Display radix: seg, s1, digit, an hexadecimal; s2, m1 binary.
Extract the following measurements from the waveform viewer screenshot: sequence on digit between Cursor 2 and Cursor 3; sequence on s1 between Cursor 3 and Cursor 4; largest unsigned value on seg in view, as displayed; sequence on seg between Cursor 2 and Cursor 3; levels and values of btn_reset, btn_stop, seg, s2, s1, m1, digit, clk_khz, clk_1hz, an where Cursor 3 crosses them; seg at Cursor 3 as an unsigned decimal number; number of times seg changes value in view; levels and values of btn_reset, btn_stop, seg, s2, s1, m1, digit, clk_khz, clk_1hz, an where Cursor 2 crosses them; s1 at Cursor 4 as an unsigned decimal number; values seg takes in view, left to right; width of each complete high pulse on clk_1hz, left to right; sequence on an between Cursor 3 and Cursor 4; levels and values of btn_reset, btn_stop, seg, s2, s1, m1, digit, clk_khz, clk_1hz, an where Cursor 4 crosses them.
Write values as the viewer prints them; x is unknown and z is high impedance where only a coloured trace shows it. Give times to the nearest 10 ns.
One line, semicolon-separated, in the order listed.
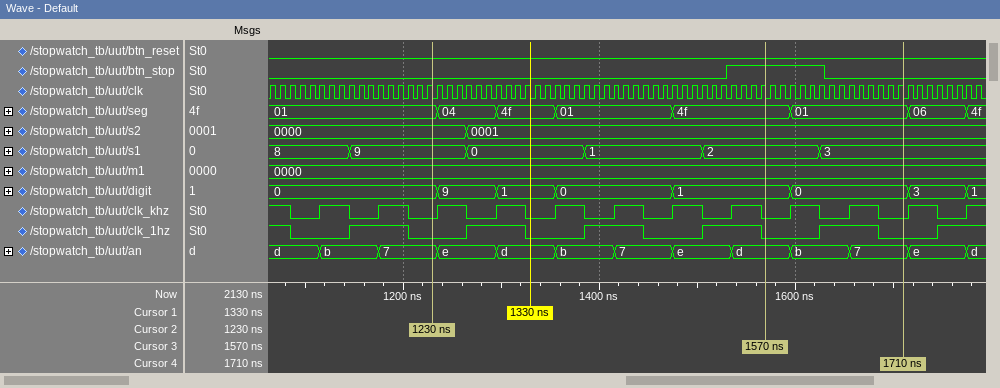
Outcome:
0, 9, 1, 0, 1; 2, 3; 4f; 01, 04, 4f, 01, 4f; btn_reset=0, btn_stop=1, seg=4f, s2=0001, s1=2, m1=0000, digit=1, clk_khz=0, clk_1hz=0, an=d; 79; 7; btn_reset=0, btn_stop=0, seg=01, s2=0000, s1=9, m1=0000, digit=0, clk_khz=0, clk_1hz=0, an=7; 3; 01, 04, 4f, 01, 4f, 01, 06, 4f; 60 ns, 60 ns, 60 ns, 60 ns, 60 ns; d, b, 7; btn_reset=0, btn_stop=0, seg=01, s2=0001, s1=3, m1=0000, digit=0, clk_khz=0, clk_1hz=0, an=7
